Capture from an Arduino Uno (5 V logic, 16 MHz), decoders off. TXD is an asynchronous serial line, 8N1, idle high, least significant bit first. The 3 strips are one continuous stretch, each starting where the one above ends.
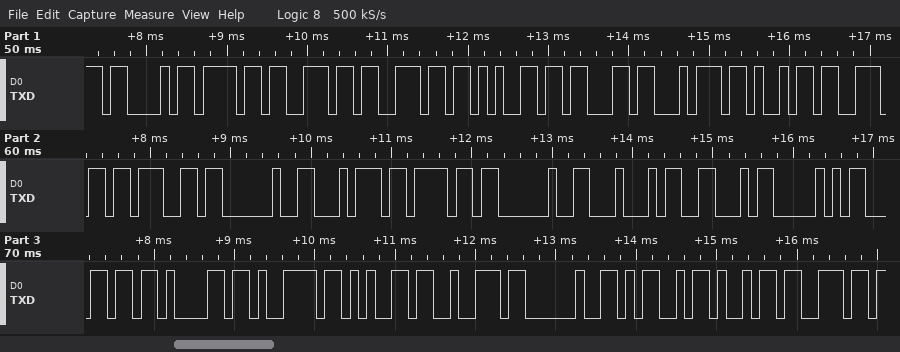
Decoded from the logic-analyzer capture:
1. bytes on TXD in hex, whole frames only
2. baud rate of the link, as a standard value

43 6F 6E 6E 65 63 74 69 6E 67 20 74 6F 20 44 46 50 6C 61 79 65 72 20 4D 69 6E
9600 baud
